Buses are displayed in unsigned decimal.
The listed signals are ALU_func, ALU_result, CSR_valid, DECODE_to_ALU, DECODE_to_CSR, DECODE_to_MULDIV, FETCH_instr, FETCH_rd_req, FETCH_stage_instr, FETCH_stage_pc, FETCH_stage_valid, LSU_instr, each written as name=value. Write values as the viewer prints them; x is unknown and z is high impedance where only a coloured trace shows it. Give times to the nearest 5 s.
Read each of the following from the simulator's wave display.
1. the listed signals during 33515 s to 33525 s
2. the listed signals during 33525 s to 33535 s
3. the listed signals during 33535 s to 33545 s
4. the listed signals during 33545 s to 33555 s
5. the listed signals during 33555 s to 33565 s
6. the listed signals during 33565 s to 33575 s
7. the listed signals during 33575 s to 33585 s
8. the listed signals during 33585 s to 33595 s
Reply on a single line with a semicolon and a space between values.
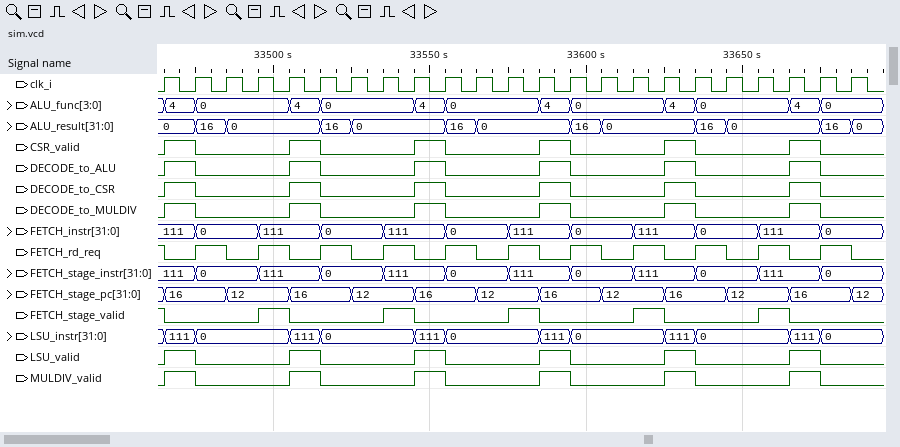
ALU_func=0, ALU_result=16, CSR_valid=0, DECODE_to_ALU=0, DECODE_to_CSR=0, DECODE_to_MULDIV=0, FETCH_instr=0, FETCH_rd_req=1, FETCH_stage_instr=0, FETCH_stage_pc=16, FETCH_stage_valid=0, LSU_instr=0; ALU_func=0, ALU_result=0, CSR_valid=0, DECODE_to_ALU=0, DECODE_to_CSR=0, DECODE_to_MULDIV=0, FETCH_instr=0, FETCH_rd_req=0, FETCH_stage_instr=0, FETCH_stage_pc=12, FETCH_stage_valid=0, LSU_instr=0; ALU_func=0, ALU_result=0, CSR_valid=0, DECODE_to_ALU=0, DECODE_to_CSR=0, DECODE_to_MULDIV=0, FETCH_instr=111, FETCH_rd_req=1, FETCH_stage_instr=111, FETCH_stage_pc=12, FETCH_stage_valid=1, LSU_instr=0; ALU_func=4, ALU_result=0, CSR_valid=1, DECODE_to_ALU=1, DECODE_to_CSR=1, DECODE_to_MULDIV=1, FETCH_instr=111, FETCH_rd_req=0, FETCH_stage_instr=111, FETCH_stage_pc=16, FETCH_stage_valid=0, LSU_instr=111; ALU_func=0, ALU_result=16, CSR_valid=0, DECODE_to_ALU=0, DECODE_to_CSR=0, DECODE_to_MULDIV=0, FETCH_instr=0, FETCH_rd_req=1, FETCH_stage_instr=0, FETCH_stage_pc=16, FETCH_stage_valid=0, LSU_instr=0; ALU_func=0, ALU_result=0, CSR_valid=0, DECODE_to_ALU=0, DECODE_to_CSR=0, DECODE_to_MULDIV=0, FETCH_instr=0, FETCH_rd_req=0, FETCH_stage_instr=0, FETCH_stage_pc=12, FETCH_stage_valid=0, LSU_instr=0; ALU_func=0, ALU_result=0, CSR_valid=0, DECODE_to_ALU=0, DECODE_to_CSR=0, DECODE_to_MULDIV=0, FETCH_instr=111, FETCH_rd_req=1, FETCH_stage_instr=111, FETCH_stage_pc=12, FETCH_stage_valid=1, LSU_instr=0; ALU_func=4, ALU_result=0, CSR_valid=1, DECODE_to_ALU=1, DECODE_to_CSR=1, DECODE_to_MULDIV=1, FETCH_instr=111, FETCH_rd_req=0, FETCH_stage_instr=111, FETCH_stage_pc=16, FETCH_stage_valid=0, LSU_instr=111
